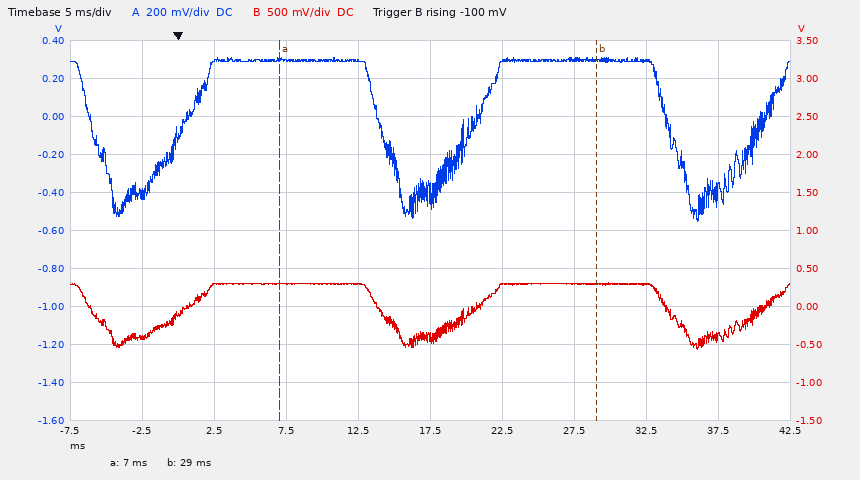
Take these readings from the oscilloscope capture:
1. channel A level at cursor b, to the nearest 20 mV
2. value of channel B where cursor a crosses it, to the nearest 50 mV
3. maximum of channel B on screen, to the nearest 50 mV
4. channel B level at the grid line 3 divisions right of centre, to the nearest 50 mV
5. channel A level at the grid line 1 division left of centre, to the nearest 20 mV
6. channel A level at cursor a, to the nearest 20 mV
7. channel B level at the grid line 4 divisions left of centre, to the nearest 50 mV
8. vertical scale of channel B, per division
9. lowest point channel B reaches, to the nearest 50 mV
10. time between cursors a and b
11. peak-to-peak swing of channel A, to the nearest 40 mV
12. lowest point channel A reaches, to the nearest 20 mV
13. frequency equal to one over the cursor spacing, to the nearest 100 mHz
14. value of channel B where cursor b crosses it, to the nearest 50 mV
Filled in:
300 mV
300 mV
300 mV
300 mV
300 mV
300 mV
-400 mV
500 mV
-550 mV
22.0 ms
880 mV
-560 mV
45.5 Hz
300 mV
